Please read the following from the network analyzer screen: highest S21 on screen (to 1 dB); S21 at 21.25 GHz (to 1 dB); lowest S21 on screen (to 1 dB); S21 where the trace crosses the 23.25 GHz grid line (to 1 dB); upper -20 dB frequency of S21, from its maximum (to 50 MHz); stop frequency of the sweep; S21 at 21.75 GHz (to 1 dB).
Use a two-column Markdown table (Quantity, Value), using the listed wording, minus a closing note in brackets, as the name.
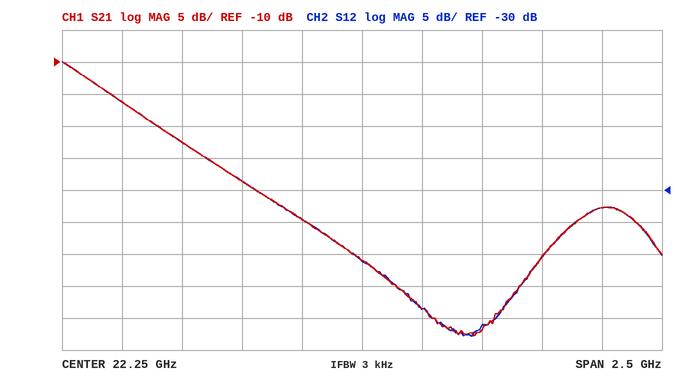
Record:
| Quantity | Value |
|---|---|
| highest S21 on screen | -10 dB |
| S21 at 21.25 GHz | -16 dB |
| lowest S21 on screen | -53 dB |
| S21 where the trace crosses the 23.25 GHz grid line | -33 dB |
| upper -20 dB frequency of S21, from its maximum | 21.80 GHz |
| stop frequency of the sweep | 23.5 GHz |
| S21 at 21.75 GHz | -29 dB |
